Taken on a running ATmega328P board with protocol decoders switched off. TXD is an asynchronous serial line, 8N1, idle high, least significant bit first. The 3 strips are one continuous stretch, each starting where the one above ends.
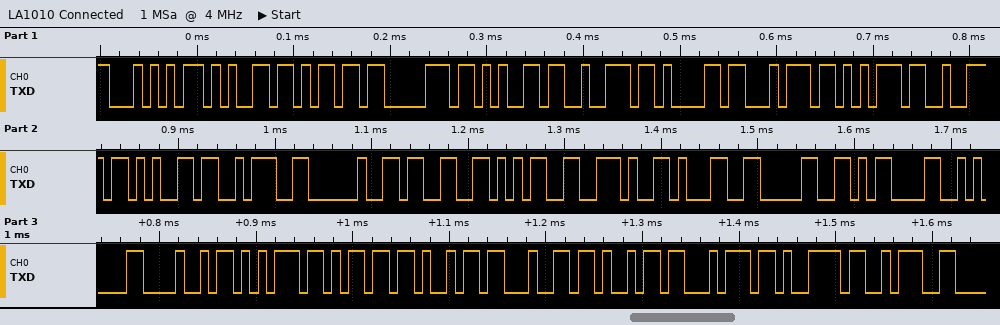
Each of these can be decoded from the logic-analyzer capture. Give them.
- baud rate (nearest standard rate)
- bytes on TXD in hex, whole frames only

115200 baud
54 65 6D 70 65 72 61 74 75 72 65 3A 20 33 35 2E 31 30 0D 0A 48 75 6D 69 64 69 74 79 3A
